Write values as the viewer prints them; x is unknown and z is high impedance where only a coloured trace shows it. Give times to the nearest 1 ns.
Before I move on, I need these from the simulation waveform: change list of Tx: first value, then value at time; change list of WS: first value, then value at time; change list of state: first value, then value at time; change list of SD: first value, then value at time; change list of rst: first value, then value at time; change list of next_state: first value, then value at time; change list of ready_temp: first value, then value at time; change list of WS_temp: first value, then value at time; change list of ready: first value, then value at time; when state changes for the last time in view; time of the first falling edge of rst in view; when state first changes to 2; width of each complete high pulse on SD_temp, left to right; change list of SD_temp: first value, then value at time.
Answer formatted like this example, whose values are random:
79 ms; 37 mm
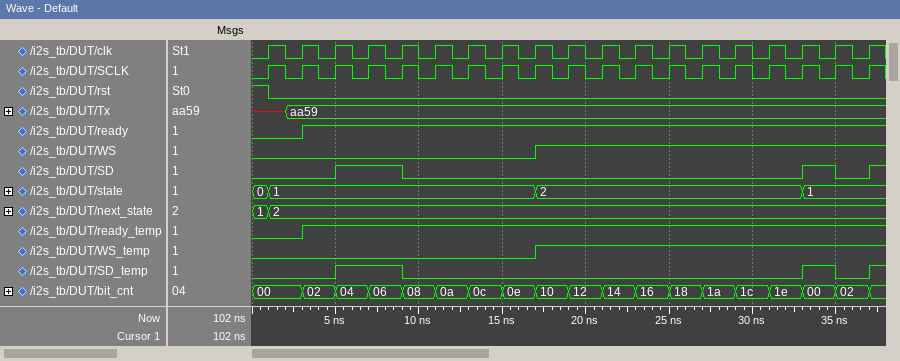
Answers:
x, aa59 at 2 ns; 0, 1 at 17 ns; 0, 1 at 1 ns, 2 at 17 ns, 1 at 33 ns; 0, 1 at 5 ns, 0 at 9 ns, 1 at 33 ns, 0 at 35 ns, 1 at 37 ns; 1, 0 at 1 ns; 1, 2 at 1 ns; 0, 1 at 3 ns; 0, 1 at 17 ns; 0, 1 at 3 ns; 33 ns; 1 ns; 17 ns; 4 ns, 2 ns; 0, 1 at 5 ns, 0 at 9 ns, 1 at 33 ns, 0 at 35 ns, 1 at 37 ns
